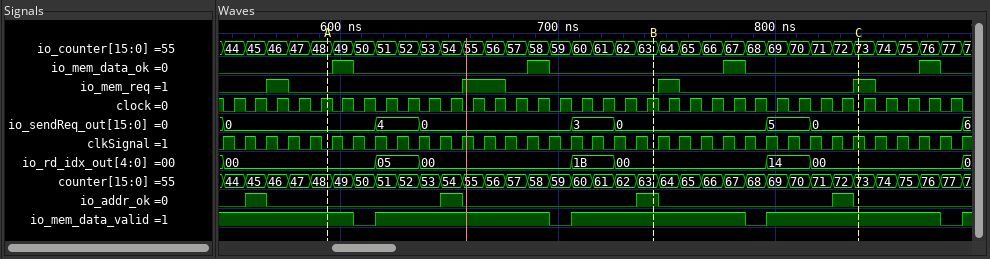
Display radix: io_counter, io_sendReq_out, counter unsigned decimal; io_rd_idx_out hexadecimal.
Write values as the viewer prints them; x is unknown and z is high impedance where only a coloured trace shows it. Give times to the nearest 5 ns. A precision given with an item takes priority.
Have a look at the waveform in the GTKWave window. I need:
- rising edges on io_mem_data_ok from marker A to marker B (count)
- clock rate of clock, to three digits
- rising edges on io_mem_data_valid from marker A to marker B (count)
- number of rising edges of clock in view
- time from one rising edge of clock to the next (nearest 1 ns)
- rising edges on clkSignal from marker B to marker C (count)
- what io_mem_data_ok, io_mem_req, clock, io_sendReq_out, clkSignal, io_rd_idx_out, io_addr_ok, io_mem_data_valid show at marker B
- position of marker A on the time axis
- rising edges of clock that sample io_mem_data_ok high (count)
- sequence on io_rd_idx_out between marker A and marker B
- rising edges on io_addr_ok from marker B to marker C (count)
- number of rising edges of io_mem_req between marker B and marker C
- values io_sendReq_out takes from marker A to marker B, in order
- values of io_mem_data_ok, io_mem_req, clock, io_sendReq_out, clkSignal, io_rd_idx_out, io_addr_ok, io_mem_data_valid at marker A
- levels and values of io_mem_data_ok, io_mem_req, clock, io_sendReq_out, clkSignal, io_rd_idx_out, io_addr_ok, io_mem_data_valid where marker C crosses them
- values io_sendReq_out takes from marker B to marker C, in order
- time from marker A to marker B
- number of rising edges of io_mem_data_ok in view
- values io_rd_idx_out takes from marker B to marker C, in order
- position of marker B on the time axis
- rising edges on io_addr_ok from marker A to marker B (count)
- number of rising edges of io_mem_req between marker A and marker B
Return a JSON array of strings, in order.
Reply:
["2", "100 MHz", "2", "34", "10 ns", "10", "io_mem_data_ok=0, io_mem_req=0, clock=1, io_sendReq_out=0, clkSignal=0, io_rd_idx_out=00, io_addr_ok=1, io_mem_data_valid=1", "595 ns", "4", "00, 05, 00, 1B, 00", "1", "2", "0, 4, 0, 3, 0", "io_mem_data_ok=0, io_mem_req=0, clock=1, io_sendReq_out=0, clkSignal=0, io_rd_idx_out=00, io_addr_ok=0, io_mem_data_valid=1", "io_mem_data_ok=0, io_mem_req=1, clock=0, io_sendReq_out=0, clkSignal=1, io_rd_idx_out=00, io_addr_ok=0, io_mem_data_valid=1", "0, 5, 0", "150 ns", "4", "00, 14, 00", "745 ns", "2", "1"]
